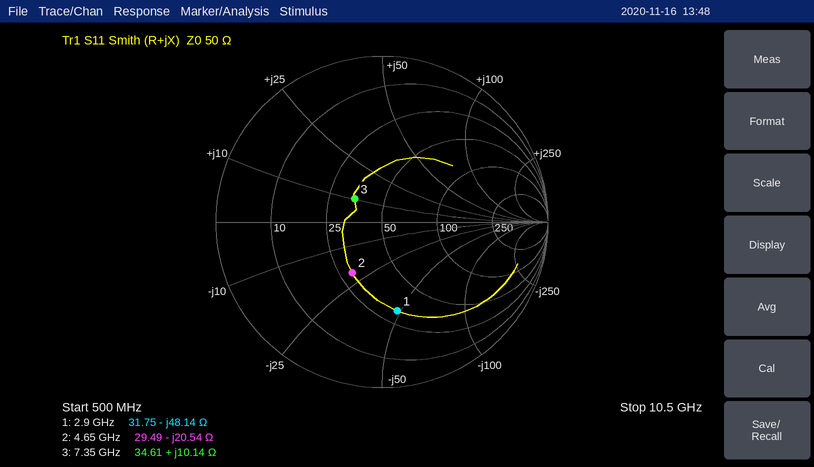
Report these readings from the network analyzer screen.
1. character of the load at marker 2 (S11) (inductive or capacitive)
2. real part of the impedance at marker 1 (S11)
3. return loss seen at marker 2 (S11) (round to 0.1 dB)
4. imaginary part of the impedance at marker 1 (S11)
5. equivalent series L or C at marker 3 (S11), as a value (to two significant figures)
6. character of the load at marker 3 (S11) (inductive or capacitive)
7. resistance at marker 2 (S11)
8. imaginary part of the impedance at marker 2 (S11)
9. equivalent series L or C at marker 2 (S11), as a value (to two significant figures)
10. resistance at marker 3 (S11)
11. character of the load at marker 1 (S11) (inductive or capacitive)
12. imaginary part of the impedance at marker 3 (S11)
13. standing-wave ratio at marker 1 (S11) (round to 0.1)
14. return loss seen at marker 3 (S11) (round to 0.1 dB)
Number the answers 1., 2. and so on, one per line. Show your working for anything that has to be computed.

1. capacitive
2. 31.75 Ω
3. 9.0 dB
4. -48.14 Ω
5. L = 10.14 Ω/(2π × 7.35 GHz) ≈ 220 pH
6. inductive
7. 29.49 Ω
8. -20.54 Ω
9. C = 1/(2π × 4.65 GHz × 20.54 Ω) ≈ 1.7 pF
10. 34.61 Ω
11. capacitive
12. +10.14 Ω
13. 3.4
14. 13.3 dB
